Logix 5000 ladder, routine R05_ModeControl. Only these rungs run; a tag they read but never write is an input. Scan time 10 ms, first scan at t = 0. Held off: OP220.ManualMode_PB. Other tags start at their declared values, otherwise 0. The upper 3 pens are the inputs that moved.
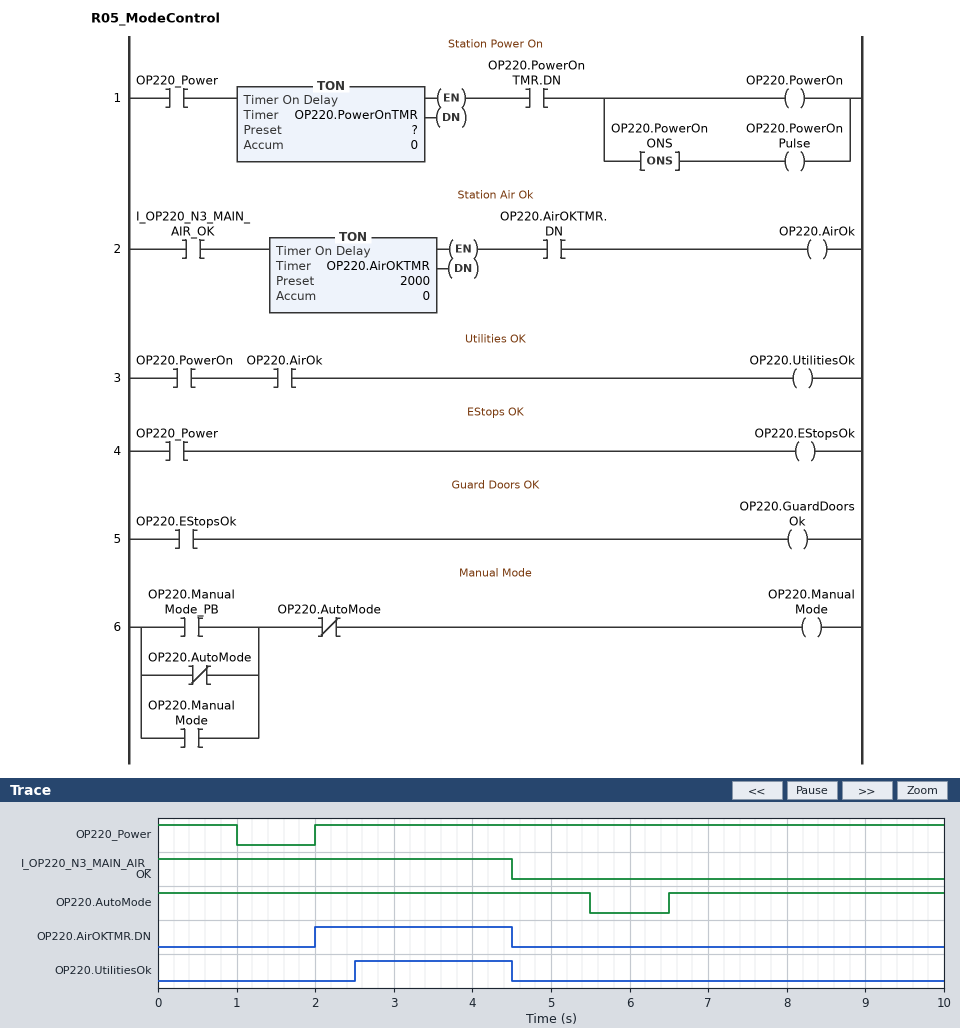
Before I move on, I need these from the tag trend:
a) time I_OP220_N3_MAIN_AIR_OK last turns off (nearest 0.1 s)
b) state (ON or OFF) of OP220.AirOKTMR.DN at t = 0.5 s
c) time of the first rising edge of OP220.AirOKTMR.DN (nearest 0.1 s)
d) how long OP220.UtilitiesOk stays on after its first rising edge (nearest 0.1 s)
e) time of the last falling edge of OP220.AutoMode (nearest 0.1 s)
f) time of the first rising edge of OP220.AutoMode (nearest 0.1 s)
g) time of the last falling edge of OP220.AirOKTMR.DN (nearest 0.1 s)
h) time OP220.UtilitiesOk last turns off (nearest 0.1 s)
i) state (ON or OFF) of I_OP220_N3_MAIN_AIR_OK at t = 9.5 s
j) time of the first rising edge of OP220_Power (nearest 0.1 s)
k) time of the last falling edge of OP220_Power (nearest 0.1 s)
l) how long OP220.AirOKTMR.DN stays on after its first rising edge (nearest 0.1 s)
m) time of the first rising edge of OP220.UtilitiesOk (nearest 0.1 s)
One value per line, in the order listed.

4.5 s
OFF
2.0 s
2.0 s
5.5 s
6.5 s
4.5 s
4.5 s
OFF
2.0 s
1.0 s
2.5 s
2.5 s
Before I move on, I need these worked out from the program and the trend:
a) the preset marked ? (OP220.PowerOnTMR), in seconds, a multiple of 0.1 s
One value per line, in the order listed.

0.5 s
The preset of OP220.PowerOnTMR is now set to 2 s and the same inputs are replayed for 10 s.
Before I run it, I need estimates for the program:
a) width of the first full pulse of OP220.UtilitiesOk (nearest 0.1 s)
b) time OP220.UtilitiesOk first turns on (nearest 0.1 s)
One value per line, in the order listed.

0.5 s
4.0 s
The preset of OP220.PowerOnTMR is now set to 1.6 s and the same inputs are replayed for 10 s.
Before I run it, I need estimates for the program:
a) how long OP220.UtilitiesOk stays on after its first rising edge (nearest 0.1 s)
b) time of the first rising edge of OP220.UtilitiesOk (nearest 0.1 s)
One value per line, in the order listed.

0.9 s
3.6 s
